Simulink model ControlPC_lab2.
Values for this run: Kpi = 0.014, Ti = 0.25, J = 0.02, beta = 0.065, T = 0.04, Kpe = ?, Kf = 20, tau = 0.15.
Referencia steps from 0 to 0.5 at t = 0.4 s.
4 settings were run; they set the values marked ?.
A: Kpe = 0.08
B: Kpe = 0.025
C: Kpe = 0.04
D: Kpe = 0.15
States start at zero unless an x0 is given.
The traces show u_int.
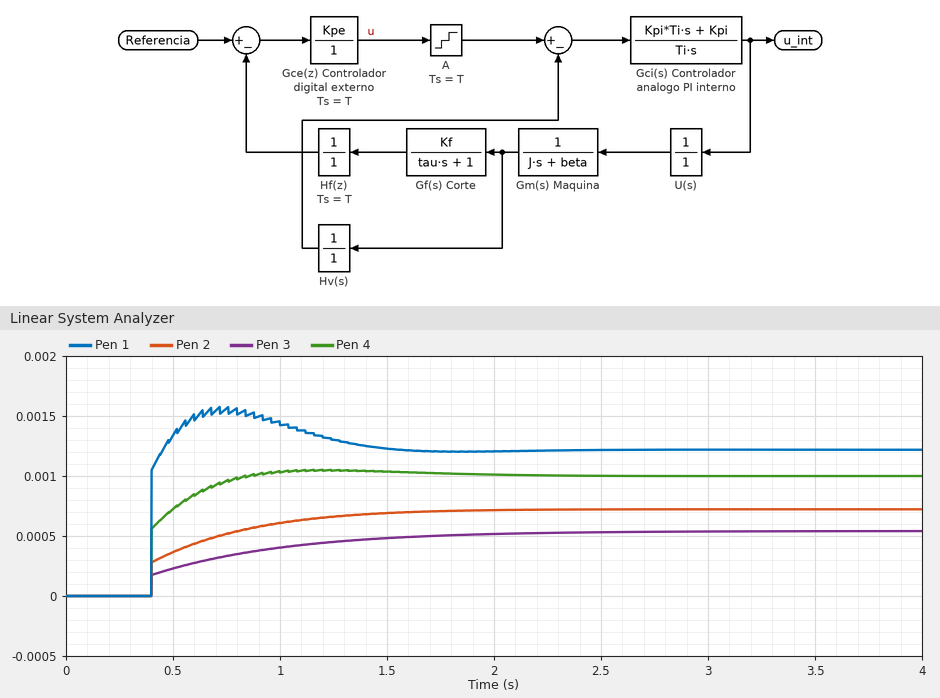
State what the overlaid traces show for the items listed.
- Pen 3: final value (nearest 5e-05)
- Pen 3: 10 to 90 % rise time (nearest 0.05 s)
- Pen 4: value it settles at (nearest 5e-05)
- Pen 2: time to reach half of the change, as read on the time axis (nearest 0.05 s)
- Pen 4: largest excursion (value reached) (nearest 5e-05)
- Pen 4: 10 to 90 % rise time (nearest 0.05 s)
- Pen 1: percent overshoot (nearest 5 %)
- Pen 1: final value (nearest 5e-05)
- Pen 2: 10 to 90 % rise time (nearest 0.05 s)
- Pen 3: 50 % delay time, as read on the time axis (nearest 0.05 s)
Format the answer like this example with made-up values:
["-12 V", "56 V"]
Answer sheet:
["0.00055", "1.15 s", "0.00100", "0.50 s", "0.00105", "0.25 s", "30 %", "0.00120", "0.80 s", "0.60 s"]
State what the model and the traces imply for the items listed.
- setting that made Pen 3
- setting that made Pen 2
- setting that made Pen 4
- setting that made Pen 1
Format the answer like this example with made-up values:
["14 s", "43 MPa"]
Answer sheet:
["B", "C", "A", "D"]
